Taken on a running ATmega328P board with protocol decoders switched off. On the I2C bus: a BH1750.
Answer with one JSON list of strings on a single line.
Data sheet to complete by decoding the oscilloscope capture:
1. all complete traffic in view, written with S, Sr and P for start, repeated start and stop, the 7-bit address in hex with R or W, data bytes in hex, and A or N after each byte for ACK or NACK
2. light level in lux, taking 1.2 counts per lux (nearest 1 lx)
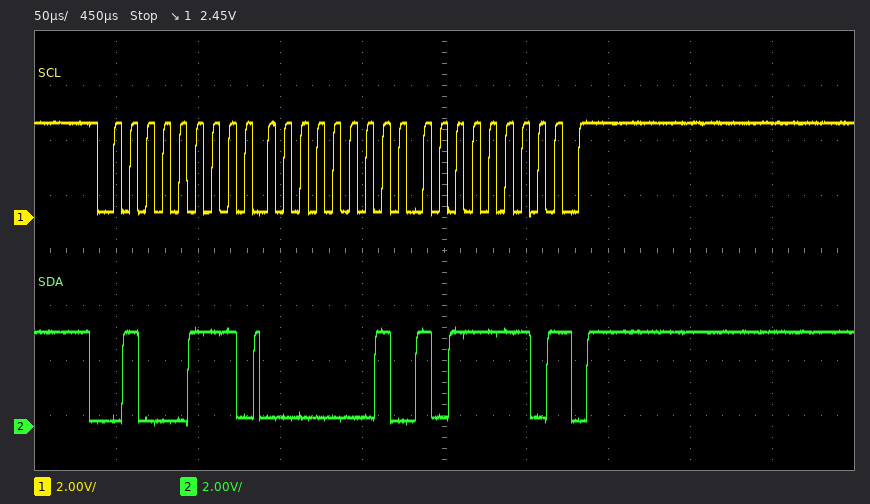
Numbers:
["S 23R A 01 A BE N P", "372 lx"]
